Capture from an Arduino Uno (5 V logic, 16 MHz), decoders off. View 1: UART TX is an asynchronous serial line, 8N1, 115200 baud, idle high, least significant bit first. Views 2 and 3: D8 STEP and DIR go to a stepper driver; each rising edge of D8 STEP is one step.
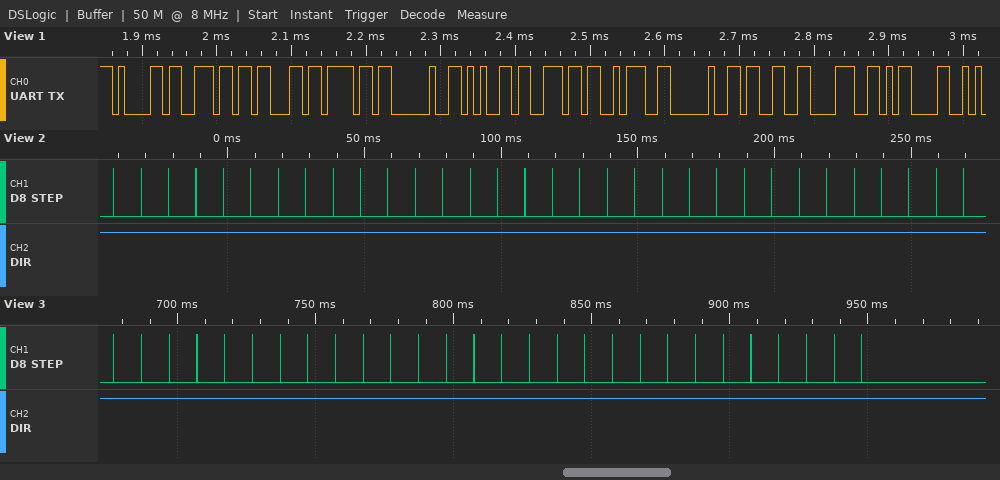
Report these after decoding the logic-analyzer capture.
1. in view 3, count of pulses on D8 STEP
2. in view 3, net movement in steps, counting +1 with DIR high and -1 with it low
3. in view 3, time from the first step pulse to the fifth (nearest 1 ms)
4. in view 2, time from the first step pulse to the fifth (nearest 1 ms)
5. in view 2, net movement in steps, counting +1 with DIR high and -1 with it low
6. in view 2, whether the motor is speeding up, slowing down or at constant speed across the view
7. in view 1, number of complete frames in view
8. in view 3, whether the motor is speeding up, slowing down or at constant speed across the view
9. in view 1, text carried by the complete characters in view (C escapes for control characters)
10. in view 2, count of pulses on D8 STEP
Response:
28
+28
40 ms
40 ms
+32
constant speed
12
constant speed
"anco en: 38\r"
32
